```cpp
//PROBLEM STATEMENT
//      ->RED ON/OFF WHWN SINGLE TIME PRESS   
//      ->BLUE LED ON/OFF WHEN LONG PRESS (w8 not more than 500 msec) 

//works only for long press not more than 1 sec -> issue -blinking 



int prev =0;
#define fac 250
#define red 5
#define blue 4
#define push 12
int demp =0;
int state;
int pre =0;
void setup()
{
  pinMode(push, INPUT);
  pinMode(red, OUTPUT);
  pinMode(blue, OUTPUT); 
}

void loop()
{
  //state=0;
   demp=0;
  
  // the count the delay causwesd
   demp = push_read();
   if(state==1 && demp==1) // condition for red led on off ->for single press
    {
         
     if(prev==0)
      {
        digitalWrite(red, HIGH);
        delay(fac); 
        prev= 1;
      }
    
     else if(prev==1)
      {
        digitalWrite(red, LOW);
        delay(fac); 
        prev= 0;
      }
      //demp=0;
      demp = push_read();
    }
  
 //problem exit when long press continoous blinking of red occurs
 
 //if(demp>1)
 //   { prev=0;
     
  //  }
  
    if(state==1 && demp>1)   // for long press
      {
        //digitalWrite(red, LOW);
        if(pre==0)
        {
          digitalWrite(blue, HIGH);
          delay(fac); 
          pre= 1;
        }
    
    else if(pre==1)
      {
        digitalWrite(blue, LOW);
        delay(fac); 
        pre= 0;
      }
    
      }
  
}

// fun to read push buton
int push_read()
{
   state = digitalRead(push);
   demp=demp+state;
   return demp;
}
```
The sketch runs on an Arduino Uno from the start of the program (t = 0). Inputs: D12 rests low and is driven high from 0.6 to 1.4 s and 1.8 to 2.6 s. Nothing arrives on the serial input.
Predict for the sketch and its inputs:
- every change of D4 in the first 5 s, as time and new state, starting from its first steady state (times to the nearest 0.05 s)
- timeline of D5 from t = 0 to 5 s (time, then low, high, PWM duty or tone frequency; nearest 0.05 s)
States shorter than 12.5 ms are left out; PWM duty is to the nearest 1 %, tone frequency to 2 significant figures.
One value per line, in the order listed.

0 s low; 0.85 s high; 1.35 s low; 2.05 s high; 2.55 s low
0 s low; 0.6 s high; 1.1 s low; 1.8 s high; 2.3 s low
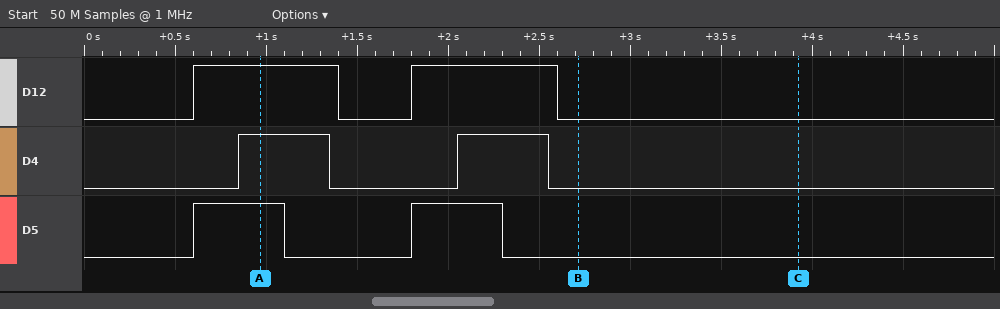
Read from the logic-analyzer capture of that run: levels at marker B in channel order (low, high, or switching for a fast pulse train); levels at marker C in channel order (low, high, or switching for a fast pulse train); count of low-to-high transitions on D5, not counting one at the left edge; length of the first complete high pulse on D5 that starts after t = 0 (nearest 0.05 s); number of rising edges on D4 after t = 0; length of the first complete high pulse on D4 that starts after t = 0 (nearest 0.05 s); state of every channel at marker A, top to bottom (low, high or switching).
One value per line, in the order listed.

D12 low, D4 low, D5 low
D12 low, D4 low, D5 low
2
0.50 s
2
0.50 s
D12 high, D4 high, D5 high
